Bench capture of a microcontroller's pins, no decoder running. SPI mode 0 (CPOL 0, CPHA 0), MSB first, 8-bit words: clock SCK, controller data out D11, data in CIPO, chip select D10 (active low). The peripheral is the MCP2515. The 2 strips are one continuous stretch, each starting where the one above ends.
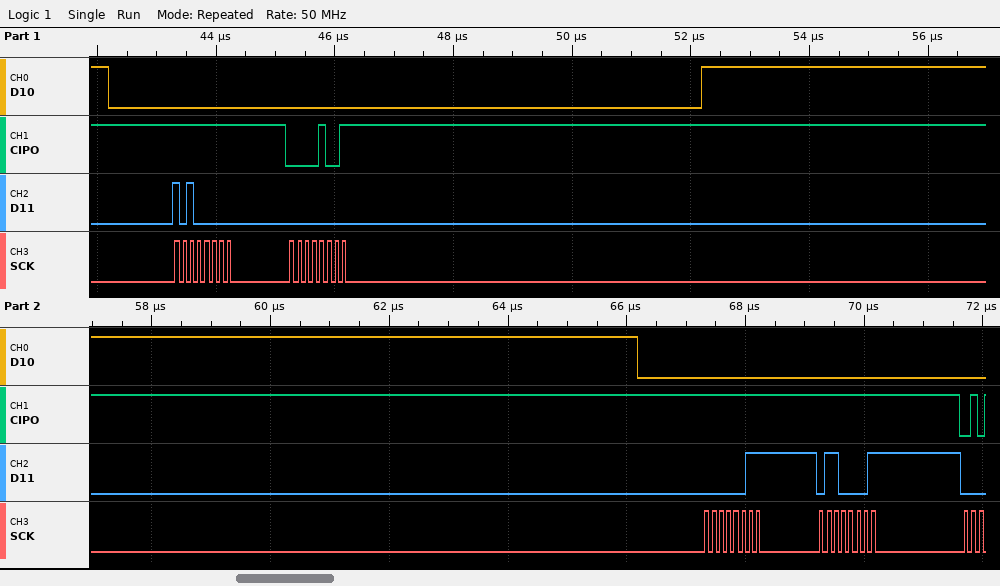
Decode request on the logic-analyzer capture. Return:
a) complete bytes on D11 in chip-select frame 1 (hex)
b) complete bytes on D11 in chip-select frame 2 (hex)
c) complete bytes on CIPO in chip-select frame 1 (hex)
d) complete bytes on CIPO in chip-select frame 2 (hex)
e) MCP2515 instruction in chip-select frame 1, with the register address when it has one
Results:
A0 00
03 61
FF 09
FF FF
READ STATUS
